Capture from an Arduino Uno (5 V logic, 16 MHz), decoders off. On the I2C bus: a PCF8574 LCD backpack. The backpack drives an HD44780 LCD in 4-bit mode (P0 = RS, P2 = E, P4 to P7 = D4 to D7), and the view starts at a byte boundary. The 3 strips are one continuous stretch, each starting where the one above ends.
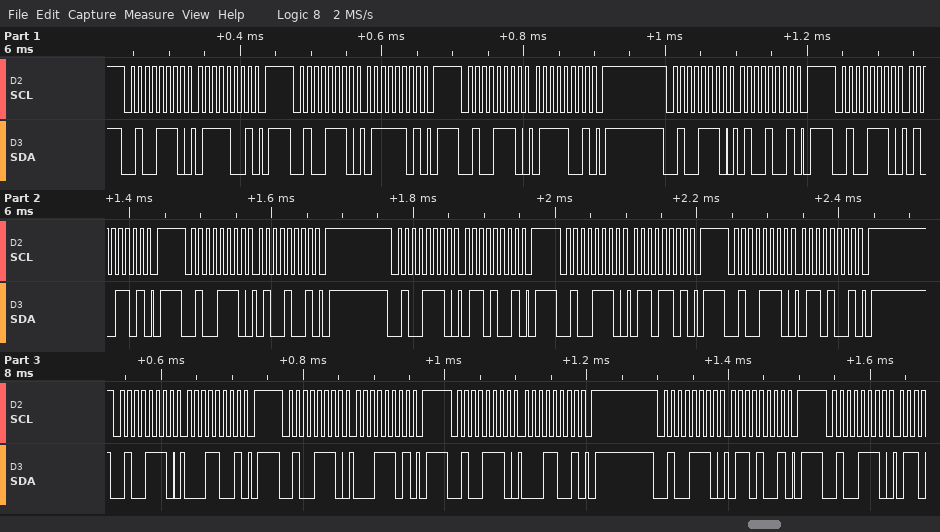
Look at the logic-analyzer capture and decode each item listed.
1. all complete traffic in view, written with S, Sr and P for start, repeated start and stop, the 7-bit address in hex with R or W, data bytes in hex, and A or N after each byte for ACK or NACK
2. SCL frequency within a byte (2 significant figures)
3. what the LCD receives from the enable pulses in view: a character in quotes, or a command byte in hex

S 27W A 79 A P S 27W A 7D A P S 27W A 79 A P S 27W A 49 A P S 27W A 4D A P S 27W A 49 A P S 27W A 69 A P S 27W A 6D A P S 27W A 69 A P S 27W A 19 A P S 27W A 1D A P S 27W A 19 A P S 27W A 69 A P S 27W A
100 kHz
't' 'a'
